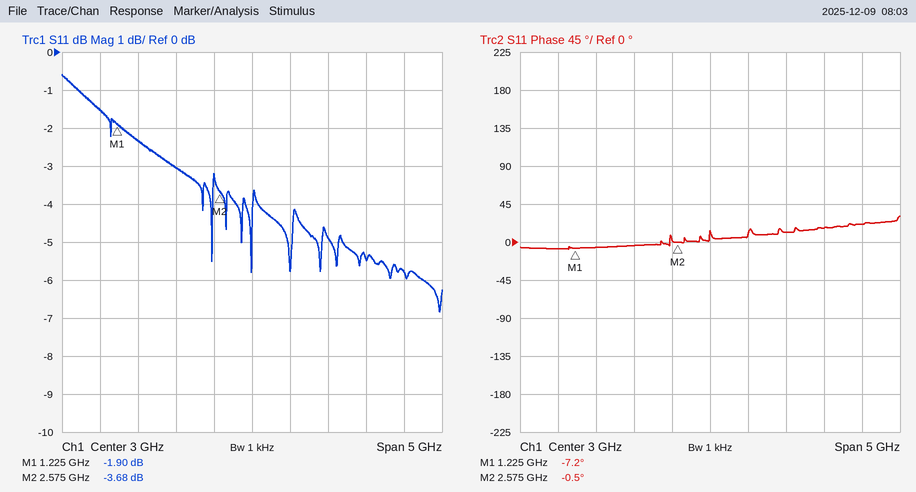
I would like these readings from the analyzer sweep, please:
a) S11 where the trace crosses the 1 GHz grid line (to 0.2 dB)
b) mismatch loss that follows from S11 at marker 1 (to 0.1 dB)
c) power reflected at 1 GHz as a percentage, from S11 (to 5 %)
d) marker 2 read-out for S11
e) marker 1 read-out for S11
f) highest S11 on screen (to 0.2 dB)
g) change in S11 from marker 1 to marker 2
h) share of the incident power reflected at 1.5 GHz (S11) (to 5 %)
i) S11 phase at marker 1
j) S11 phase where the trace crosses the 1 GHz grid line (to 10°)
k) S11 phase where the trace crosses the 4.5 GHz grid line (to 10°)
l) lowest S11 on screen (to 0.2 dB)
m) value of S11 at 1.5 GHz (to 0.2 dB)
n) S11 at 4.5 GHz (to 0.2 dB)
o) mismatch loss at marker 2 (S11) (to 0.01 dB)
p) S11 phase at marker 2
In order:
-1.6 dB
4.5 dB
70 %
-3.68 dB
-1.90 dB
-0.6 dB
-1.78 dB
60 %
-7.2°
-10°
20°
-6.8 dB
-2.4 dB
-5.4 dB
2.43 dB
-0.5°
